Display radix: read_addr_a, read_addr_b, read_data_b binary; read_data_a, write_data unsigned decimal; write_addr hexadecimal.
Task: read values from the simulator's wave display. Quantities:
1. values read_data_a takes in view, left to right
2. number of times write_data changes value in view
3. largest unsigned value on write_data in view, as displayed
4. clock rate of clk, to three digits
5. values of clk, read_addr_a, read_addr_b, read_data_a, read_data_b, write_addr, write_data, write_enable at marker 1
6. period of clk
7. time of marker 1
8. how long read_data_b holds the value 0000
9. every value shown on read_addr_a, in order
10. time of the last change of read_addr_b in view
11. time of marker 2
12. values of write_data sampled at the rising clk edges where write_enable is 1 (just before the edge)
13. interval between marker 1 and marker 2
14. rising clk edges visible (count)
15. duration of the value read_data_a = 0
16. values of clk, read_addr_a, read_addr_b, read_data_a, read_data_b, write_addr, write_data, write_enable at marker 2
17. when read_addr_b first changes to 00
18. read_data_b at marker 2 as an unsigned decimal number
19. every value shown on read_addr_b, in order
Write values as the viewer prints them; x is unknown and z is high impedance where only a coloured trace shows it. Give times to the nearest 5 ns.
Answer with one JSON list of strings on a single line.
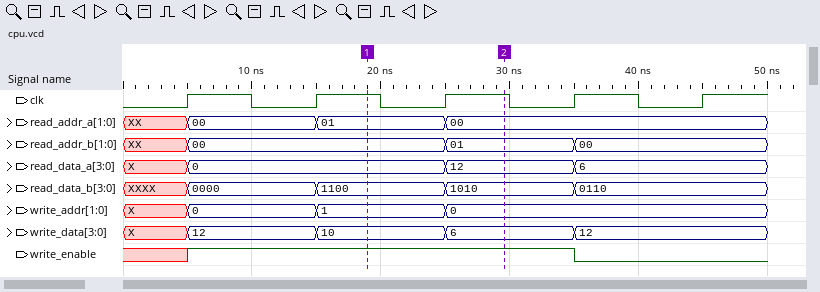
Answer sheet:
["X, 0, 12, 6", "4", "12", "100 MHz", "clk=1, read_addr_a=01, read_addr_b=00, read_data_a=0, read_data_b=1100, write_addr=1, write_data=10, write_enable=1", "10 ns", "20 ns", "10 ns", "XX, 00, 01, 00", "35 ns", "30 ns", "12, 10, 6", "10 ns", "5", "20 ns", "clk=1, read_addr_a=00, read_addr_b=01, read_data_a=12, read_data_b=1010, write_addr=0, write_data=6, write_enable=1", "5 ns", "10", "XX, 00, 01, 00"]
